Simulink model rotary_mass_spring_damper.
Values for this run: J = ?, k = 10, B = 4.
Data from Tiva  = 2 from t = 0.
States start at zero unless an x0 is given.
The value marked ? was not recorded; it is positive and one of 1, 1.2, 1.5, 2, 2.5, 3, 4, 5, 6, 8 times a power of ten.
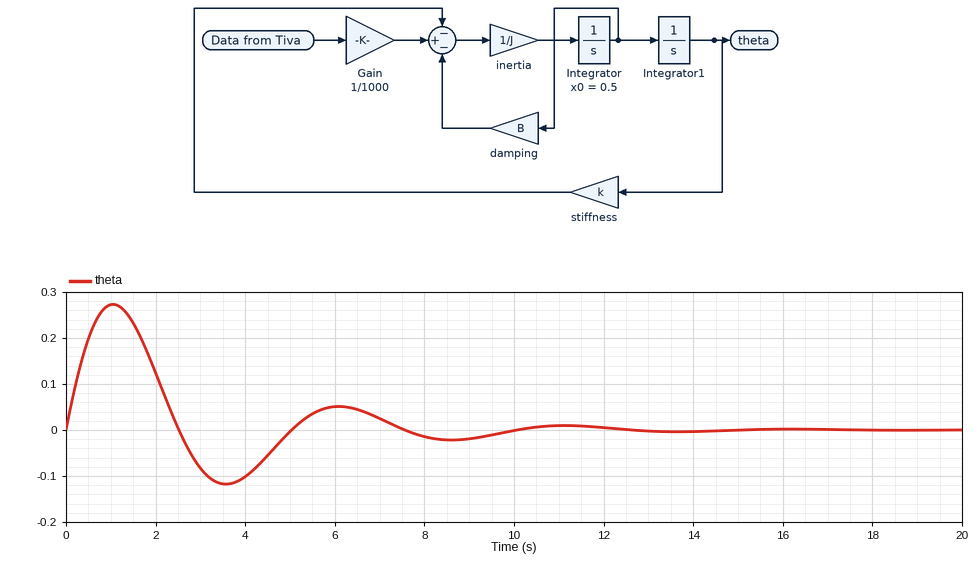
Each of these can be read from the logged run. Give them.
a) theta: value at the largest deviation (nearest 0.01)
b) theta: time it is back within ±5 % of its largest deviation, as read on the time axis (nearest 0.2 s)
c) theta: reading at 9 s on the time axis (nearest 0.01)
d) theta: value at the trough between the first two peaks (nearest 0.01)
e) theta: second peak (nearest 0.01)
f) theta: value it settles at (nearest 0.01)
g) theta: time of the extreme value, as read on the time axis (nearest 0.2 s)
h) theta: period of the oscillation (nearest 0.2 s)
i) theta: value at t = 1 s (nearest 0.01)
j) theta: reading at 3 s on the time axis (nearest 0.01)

0.27
9.4 s
-0.02
-0.12
0.05
0.00
1.0 s
5.0 s
0.27
-0.08
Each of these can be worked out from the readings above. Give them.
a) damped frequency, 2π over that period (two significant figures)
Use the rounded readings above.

1.3 rad/s
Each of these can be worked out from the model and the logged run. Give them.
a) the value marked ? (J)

6
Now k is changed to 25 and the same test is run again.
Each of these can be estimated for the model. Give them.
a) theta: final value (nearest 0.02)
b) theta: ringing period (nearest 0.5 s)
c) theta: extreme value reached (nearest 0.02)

0.00
3.0 s
0.20
